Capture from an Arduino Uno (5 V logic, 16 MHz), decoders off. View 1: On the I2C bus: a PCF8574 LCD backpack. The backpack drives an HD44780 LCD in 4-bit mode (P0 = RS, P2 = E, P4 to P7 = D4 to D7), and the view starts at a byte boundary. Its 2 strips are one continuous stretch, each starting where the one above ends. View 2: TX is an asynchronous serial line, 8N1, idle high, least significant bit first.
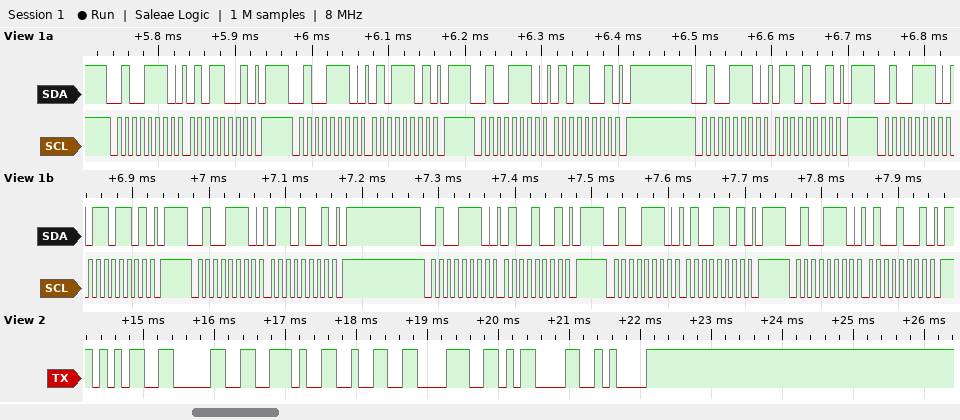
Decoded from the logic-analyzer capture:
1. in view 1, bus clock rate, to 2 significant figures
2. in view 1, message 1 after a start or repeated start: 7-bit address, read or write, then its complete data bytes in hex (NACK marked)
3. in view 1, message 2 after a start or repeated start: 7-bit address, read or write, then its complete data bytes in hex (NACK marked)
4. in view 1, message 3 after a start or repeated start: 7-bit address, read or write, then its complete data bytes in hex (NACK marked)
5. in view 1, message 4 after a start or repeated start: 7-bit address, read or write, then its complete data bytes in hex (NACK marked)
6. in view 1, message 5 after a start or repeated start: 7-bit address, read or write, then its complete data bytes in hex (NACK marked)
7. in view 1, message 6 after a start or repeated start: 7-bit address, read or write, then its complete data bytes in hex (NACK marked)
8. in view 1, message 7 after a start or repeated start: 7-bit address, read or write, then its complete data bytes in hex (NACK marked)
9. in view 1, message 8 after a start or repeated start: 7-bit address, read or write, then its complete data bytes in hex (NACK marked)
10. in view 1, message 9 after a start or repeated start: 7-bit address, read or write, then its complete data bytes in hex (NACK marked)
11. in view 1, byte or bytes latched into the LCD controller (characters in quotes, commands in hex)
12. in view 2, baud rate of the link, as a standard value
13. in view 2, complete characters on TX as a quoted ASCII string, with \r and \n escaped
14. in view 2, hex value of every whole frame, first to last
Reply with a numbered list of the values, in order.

1. 100 kHz
2. 0x27 write: 59
3. 0x27 write: 5D
4. 0x27 write: 59
5. 0x27 write: 69
6. 0x27 write: 6D
7. 0x27 write: 69
8. 0x27 write: 49
9. 0x27 write: 4D
10. 0x27 write: 49
11. 'V'
12. 9600 baud
13. "50.28\r\n"
14. 35 30 2E 32 38 0D 0A
